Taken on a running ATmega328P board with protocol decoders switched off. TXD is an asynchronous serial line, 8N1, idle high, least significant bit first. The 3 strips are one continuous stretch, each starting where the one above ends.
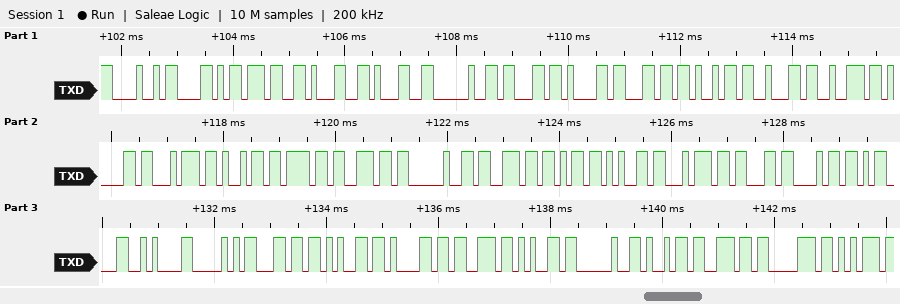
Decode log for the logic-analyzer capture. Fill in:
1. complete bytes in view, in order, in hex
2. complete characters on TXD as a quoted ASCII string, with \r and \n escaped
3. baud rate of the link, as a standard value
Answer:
0x48 0x58 0x37 0x31 0x31 0x20 0x63 0x61 0x6C 0x69 0x62 0x72 0x61 0x74 0x69 0x6F 0x6E 0x20 0x73 0x6B 0x65 0x74 0x63 0x68 0x0D 0x0A 0x50 0x6C 0x65 0x61 0x73 0x65 0x20 0x69 0x6E 0x70 0x75
"HX711 calibration sketch\r\nPlease inpu"
9600 baud
